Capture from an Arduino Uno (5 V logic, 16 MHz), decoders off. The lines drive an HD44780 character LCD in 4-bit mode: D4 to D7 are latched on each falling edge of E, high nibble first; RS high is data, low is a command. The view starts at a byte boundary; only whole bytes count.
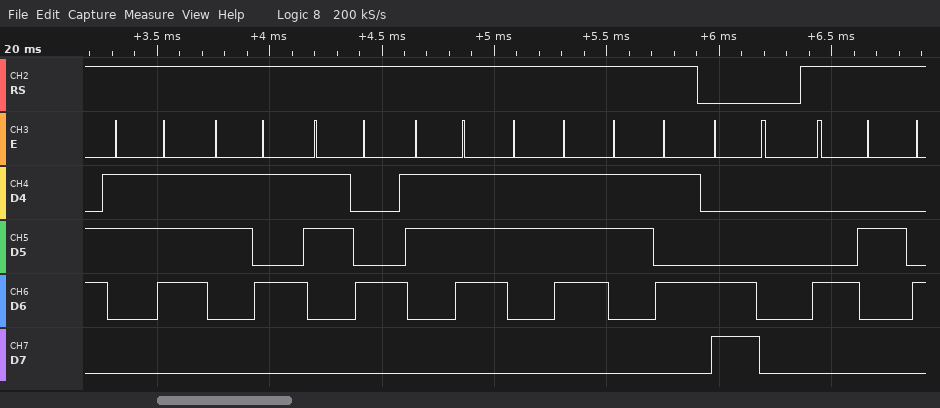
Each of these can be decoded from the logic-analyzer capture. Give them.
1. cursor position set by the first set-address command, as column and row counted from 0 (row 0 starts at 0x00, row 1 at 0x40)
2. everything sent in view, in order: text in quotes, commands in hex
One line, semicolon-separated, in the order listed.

column 0, row 1; "754775" 0xC0 "B"
